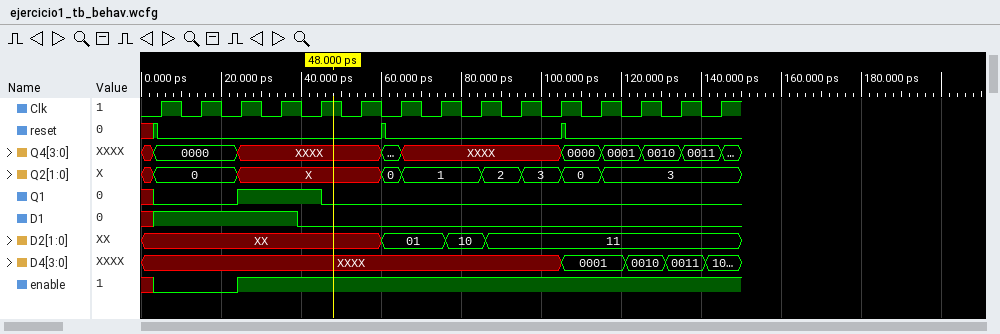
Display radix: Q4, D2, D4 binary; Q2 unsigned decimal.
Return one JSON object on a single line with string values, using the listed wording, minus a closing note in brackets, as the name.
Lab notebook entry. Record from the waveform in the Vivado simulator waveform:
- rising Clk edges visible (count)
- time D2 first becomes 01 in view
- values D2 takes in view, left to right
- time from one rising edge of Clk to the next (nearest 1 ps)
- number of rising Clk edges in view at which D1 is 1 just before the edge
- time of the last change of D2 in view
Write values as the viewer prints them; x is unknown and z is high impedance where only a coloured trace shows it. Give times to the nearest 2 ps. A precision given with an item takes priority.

{"rising Clk edges visible": "15", "time D2 first becomes 01 in view": "60 ps", "values D2 takes in view, left to right": "XX, 01, 10, 11", "time from one rising edge of Clk to the next": "10 ps", "number of rising Clk edges in view at which D1 is 1 just before the edge": "4", "time of the last change of D2 in view": "86 ps"}
